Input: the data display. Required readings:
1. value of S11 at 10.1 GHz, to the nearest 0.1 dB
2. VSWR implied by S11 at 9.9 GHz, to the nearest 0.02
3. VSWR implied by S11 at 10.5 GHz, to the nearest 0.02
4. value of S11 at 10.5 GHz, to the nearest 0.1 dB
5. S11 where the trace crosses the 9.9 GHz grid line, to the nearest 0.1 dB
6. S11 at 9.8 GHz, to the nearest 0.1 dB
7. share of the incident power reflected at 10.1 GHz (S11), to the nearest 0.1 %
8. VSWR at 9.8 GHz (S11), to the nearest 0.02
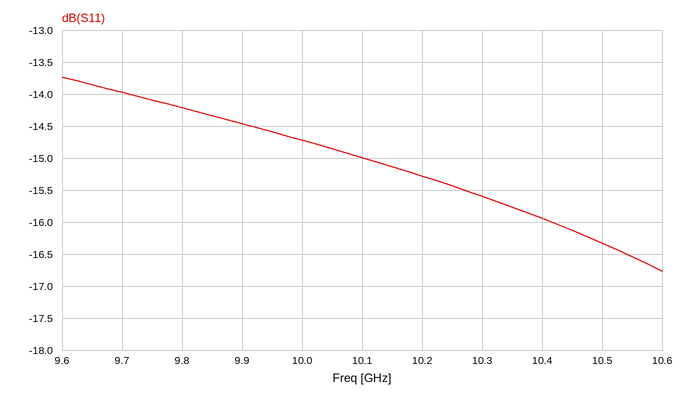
-15.0 dB
1.46
1.36
-16.3 dB
-14.5 dB
-14.2 dB
3.2 %
1.48
